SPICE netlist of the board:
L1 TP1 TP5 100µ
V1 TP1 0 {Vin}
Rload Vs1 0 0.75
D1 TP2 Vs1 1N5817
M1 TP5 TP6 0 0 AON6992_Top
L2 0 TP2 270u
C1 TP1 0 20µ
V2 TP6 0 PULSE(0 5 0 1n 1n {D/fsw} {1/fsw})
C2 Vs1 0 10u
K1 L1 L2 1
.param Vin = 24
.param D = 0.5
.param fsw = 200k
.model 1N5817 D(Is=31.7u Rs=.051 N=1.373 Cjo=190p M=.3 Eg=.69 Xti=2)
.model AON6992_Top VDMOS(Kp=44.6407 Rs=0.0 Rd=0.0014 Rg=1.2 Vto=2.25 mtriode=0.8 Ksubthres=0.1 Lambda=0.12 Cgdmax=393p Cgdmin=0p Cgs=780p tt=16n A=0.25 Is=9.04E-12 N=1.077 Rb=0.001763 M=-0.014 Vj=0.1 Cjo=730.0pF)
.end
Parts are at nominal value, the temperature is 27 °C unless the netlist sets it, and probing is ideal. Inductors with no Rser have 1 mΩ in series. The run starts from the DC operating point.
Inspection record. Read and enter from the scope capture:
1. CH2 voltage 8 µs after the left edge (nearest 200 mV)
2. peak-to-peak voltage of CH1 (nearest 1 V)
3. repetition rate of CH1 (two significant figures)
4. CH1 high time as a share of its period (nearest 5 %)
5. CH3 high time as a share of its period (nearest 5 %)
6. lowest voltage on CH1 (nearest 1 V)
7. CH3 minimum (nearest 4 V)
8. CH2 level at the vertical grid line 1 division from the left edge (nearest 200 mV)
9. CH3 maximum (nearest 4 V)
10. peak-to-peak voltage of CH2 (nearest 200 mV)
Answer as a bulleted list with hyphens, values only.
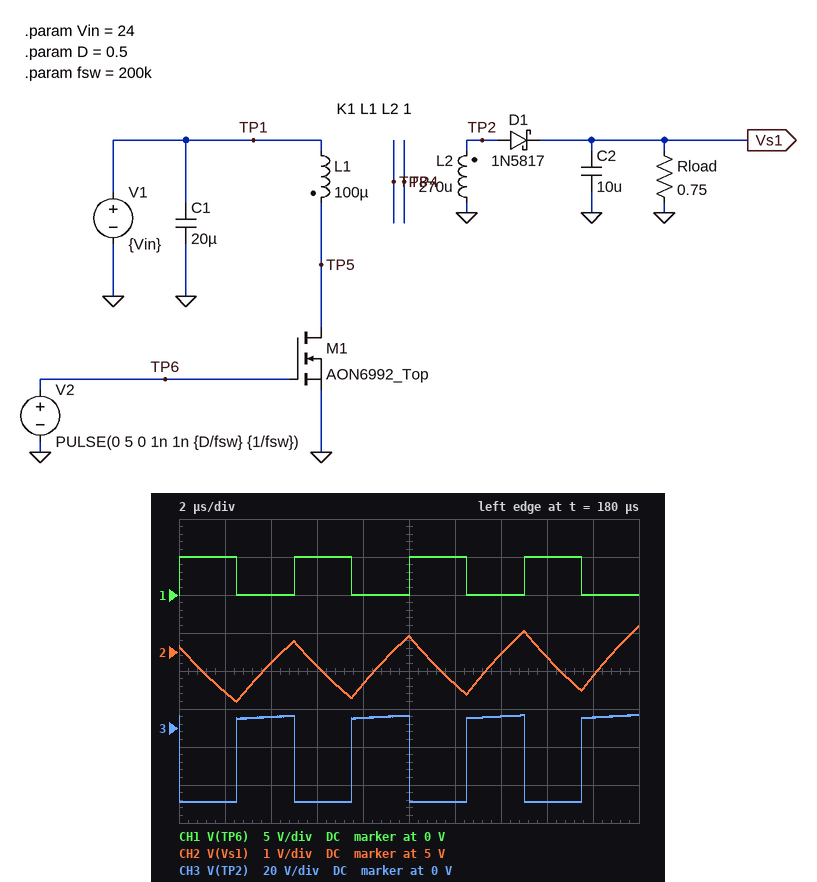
- 4.2 V
- 5 V
- 200 kHz
- 50 %
- 50 %
- 0 V
- -40 V
- 4.0 V
- 8 V
- 2.0 V
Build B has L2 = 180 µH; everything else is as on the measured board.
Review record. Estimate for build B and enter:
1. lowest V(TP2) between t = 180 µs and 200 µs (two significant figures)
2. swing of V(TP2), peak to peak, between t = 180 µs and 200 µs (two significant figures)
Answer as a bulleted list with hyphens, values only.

- -32 V
- 40 V
